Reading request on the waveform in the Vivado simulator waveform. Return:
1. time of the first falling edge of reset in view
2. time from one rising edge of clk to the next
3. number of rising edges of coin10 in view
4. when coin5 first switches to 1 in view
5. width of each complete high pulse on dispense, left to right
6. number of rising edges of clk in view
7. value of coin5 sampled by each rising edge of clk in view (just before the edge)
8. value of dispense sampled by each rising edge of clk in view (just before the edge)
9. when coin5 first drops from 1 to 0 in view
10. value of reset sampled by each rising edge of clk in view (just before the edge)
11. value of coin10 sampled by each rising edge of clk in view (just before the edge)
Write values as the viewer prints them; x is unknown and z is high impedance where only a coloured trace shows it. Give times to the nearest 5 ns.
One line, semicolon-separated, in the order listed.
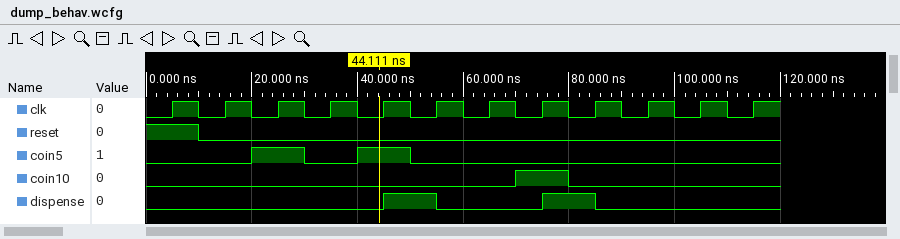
10 ns; 10 ns; 1; 20 ns; 10 ns, 10 ns; 12; 0 0 1 0 1 0 0 0 0 0 0 0; 0 0 0 0 0 1 0 0 1 0 0 0; 30 ns; 1 0 0 0 0 0 0 0 0 0 0 0; 0 0 0 0 0 0 0 1 0 0 0 0
